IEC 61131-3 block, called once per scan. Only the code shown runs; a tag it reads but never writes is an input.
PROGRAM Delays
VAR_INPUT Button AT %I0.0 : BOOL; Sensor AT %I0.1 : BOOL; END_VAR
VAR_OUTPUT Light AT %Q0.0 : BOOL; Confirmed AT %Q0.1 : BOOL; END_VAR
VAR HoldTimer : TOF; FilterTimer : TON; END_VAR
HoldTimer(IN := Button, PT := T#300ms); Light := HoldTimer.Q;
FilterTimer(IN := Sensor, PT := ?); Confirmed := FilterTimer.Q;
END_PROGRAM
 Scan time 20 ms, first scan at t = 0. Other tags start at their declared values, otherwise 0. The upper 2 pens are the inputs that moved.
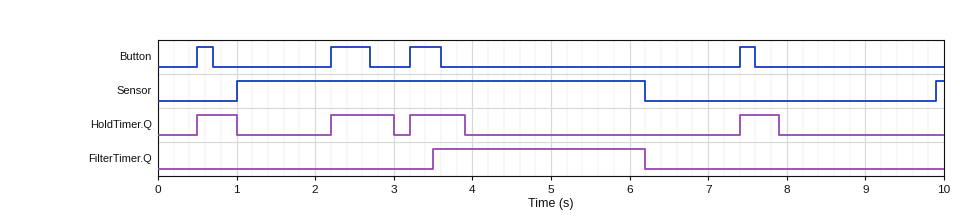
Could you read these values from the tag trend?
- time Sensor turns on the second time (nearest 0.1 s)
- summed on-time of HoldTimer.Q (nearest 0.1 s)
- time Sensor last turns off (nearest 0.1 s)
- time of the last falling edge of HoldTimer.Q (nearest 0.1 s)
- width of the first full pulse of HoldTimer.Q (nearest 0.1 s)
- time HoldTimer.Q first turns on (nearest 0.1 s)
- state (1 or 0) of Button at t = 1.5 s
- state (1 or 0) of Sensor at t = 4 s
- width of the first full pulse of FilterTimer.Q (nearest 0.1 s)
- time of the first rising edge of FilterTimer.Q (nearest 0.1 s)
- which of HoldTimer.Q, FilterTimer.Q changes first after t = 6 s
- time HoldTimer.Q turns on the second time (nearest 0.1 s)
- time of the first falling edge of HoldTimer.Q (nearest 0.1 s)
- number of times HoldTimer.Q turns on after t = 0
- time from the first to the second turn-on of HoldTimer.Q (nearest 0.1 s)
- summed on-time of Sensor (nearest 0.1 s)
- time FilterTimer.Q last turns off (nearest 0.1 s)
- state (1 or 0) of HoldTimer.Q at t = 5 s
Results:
9.9 s
2.5 s
6.2 s
7.9 s
0.5 s
0.5 s
0
1
2.7 s
3.5 s
FilterTimer.Q
2.2 s
1.0 s
4
1.7 s
5.3 s
6.2 s
0
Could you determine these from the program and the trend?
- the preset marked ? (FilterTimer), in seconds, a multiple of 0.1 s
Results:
2.5 s
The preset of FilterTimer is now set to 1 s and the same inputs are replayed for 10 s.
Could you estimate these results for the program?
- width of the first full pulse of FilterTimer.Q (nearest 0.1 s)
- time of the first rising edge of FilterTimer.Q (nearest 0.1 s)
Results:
4.2 s
2.0 s
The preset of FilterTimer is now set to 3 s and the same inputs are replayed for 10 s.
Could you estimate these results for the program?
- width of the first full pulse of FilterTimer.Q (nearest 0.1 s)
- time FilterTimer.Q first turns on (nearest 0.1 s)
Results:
2.2 s
4.0 s
